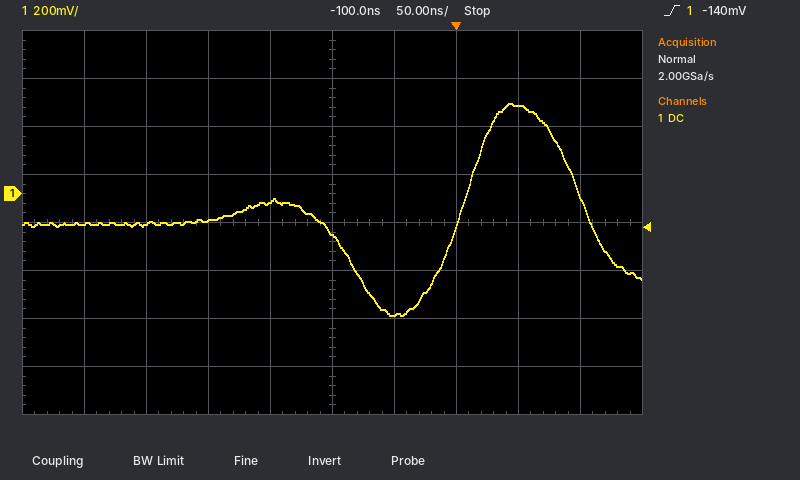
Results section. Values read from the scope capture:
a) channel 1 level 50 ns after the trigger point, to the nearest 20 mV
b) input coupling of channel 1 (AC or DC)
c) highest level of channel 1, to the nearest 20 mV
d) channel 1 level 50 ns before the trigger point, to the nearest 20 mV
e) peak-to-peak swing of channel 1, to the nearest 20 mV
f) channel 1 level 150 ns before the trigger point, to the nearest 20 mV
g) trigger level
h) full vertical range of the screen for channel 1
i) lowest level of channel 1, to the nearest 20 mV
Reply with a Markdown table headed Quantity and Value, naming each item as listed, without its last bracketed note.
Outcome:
| Quantity | Value |
|---|---|
| channel 1 level 50 ns after the trigger point, to the nearest 20 mV | 360 mV |
| input coupling of channel 1 | DC |
| highest level of channel 1, to the nearest 20 mV | 380 mV |
| channel 1 level 50 ns before the trigger point, to the nearest 20 mV | -500 mV |
| peak-to-peak swing of channel 1, to the nearest 20 mV | 880 mV |
| channel 1 level 150 ns before the trigger point, to the nearest 20 mV | -40 mV |
| trigger level | -140 mV |
| full vertical range of the screen for channel 1 | 1.6 V |
| lowest level of channel 1, to the nearest 20 mV | -500 mV |
